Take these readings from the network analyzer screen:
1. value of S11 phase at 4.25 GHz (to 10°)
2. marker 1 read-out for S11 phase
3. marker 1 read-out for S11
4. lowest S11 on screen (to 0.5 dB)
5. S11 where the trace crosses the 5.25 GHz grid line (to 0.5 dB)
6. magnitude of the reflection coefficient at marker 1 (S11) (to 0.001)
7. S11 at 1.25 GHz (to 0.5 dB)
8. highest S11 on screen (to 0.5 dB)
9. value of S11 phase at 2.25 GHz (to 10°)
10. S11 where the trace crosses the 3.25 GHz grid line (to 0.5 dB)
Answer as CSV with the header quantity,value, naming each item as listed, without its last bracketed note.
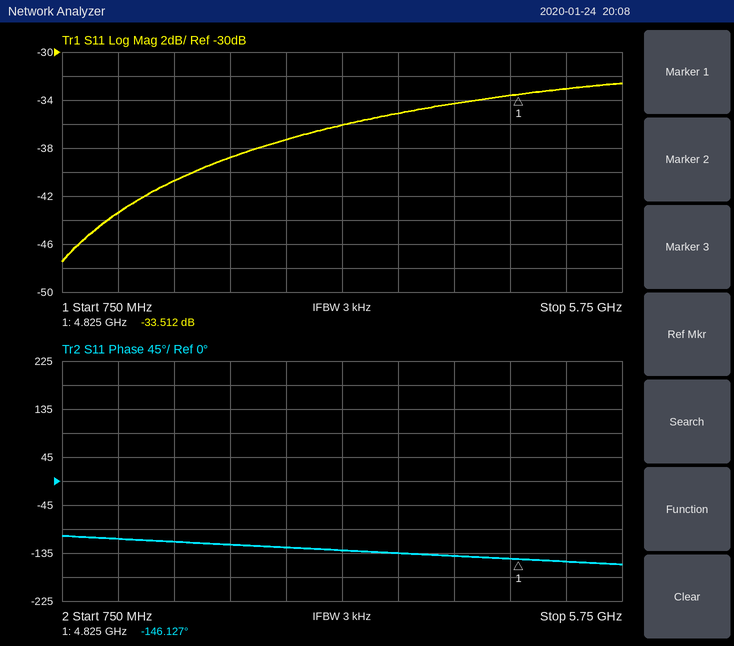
quantity,value
value of S11 phase at 4.25 GHz,-140°
marker 1 read-out for S11 phase,-146.127°
marker 1 read-out for S11,-33.512 dB
lowest S11 on screen,-47.5 dB
S11 where the trace crosses the 5.25 GHz grid line,-33.0 dB
magnitude of the reflection coefficient at marker 1 (S11),0.021
S11 at 1.25 GHz,-43.5 dB
highest S11 on screen,-32.5 dB
value of S11 phase at 2.25 GHz,-120°
S11 where the trace crosses the 3.25 GHz grid line,-36.0 dB
